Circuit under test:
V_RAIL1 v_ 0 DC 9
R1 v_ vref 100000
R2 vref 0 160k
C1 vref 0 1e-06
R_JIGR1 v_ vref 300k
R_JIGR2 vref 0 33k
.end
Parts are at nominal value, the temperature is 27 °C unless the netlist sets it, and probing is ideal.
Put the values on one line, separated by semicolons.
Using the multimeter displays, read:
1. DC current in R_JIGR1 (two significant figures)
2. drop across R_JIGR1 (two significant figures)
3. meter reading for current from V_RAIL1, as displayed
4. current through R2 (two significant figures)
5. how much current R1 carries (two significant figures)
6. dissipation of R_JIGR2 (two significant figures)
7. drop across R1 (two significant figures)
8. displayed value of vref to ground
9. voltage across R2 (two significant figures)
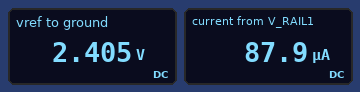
22 µA; 6.6 V; 87.9 µA; 15 µA; 66 µA; 180 µW; 6.6 V; 2.405 V; 2.4 V
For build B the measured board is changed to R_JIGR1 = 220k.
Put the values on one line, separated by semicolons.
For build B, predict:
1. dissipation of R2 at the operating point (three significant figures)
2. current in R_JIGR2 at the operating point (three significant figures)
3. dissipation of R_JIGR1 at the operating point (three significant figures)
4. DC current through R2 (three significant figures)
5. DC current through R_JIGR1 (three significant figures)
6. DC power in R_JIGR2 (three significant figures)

41.0 µW; 77.6 µA; 188 µW; 16.0 µA; 29.3 µA; 199 µW
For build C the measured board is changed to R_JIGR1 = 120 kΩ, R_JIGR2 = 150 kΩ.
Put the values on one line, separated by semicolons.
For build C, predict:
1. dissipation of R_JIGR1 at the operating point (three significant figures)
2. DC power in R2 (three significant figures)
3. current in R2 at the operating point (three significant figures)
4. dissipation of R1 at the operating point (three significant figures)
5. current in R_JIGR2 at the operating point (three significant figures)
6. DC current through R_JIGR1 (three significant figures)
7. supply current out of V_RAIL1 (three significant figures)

115 µW; 174 µW; 33.0 µA; 138 µW; 35.2 µA; 31.0 µA; 68.2 µA
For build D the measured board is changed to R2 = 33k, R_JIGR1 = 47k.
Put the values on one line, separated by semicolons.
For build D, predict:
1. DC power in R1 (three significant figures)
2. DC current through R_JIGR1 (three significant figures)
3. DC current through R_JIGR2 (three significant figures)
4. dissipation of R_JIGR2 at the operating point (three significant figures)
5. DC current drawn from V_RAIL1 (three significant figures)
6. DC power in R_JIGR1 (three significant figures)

352 µW; 126 µA; 92.8 µA; 284 µW; 186 µA; 750 µW
